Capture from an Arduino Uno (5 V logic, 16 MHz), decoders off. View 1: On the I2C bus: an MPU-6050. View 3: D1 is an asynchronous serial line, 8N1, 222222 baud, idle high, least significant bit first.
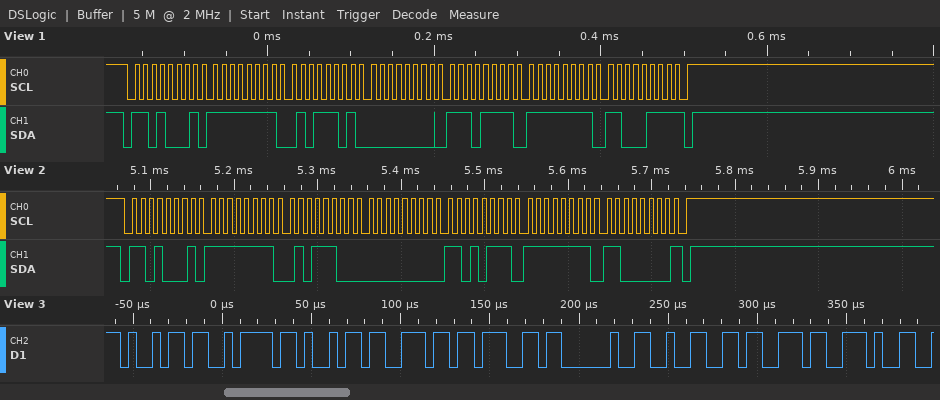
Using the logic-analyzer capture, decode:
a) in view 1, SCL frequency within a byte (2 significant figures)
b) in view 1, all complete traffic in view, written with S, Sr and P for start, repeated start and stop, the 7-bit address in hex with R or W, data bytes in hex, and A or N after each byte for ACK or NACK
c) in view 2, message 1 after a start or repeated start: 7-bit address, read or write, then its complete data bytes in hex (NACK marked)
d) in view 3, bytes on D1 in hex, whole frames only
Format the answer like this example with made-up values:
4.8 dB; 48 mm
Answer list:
100 kHz; S 68R A FF A 5D A 00 A EF A FF A C7 N P; 0x68 read: FF 5C 00 D7 FF C0 NACK; 69 7A 69 6E 67 20 32 73 2E
